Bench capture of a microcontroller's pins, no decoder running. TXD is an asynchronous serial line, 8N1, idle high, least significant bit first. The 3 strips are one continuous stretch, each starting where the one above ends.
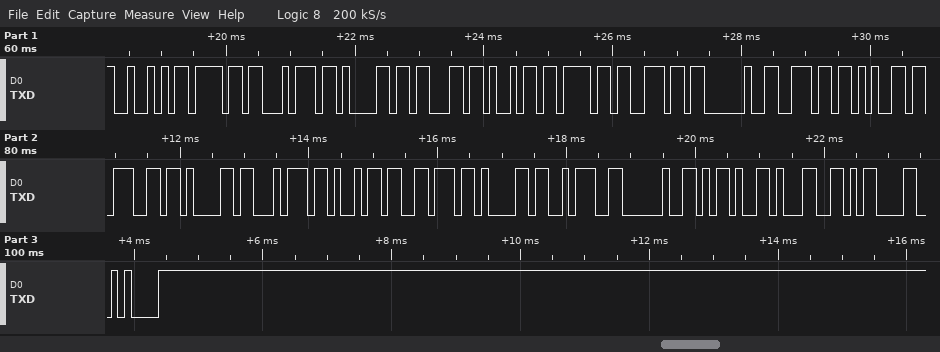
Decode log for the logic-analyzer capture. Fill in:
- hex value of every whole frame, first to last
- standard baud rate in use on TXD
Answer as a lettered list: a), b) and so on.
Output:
a) 52 6F 74 61 63 69 6F 6E 20 6E 65 67 61 74 69 76 61 3A 20 2D 31 0D 0A
b) 9600 baud
